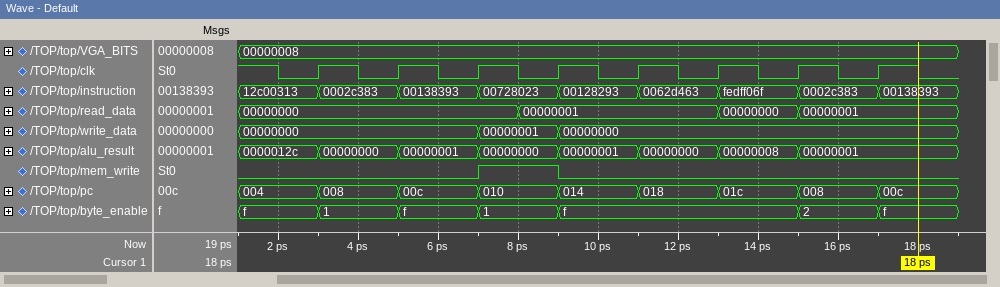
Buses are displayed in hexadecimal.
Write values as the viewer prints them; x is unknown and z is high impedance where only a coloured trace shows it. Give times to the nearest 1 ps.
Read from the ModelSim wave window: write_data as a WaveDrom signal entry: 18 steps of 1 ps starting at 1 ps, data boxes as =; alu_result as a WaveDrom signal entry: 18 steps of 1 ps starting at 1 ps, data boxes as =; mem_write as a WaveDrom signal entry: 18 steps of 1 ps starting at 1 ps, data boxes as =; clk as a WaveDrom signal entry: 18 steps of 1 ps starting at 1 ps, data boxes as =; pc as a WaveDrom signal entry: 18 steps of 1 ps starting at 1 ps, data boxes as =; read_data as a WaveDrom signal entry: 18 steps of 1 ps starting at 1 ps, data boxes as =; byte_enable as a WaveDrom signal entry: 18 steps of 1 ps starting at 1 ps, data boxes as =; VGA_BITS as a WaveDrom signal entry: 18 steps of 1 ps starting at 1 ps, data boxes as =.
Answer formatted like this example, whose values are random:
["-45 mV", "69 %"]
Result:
["{name: 'write_data', wave: '=.....=.=.........', data: '00000000 00000001 00000000'}", "{name: 'alu_result', wave: '=.=.=.=.=.=.=.=...', data: '0000012c 00000000 00000001 00000000 00000001 00000000 00000008 00000001'}", "{name: 'mem_write', wave: '0.....1.0.........'}", "{name: 'clk', wave: '101010101010101010'}", "{name: 'pc', wave: '=.=.=.=.=.=.=.=.=.', data: '004 008 00c 010 014 018 01c 008 00c'}", "{name: 'read_data', wave: '=......=....=.=...', data: '00000000 00000001 00000000 00000001'}", "{name: 'byte_enable', wave: '=.=.=.=.=.....=.=.', data: 'f 1 f 1 f 2 f'}", "{name: 'VGA_BITS', wave: '=.................', data: '00000008'}"]
